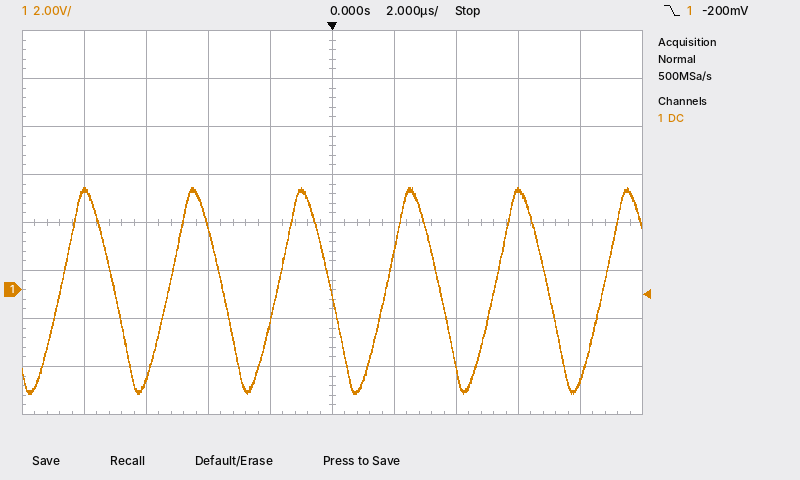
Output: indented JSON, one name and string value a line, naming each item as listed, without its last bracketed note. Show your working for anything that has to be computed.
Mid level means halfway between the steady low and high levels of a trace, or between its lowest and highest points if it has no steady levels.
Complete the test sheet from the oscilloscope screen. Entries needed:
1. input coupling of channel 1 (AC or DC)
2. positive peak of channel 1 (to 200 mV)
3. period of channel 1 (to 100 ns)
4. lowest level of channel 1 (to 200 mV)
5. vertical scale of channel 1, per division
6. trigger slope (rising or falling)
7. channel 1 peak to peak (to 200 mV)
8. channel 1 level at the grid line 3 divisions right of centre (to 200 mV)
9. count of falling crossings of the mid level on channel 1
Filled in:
{
  "input coupling of channel 1": "DC",
  "positive peak of channel 1": "4.2 V",
  "period of channel 1": "3.5 µs",
  "lowest level of channel 1": "-4.4 V",
  "vertical scale of channel 1, per division": "2 V",
  "trigger slope": "falling",
  "channel 1 peak to peak": "4.2 V − (-4.4 V) = 8.6 V",
  "channel 1 level at the grid line 3 divisions right of centre": "4.2 V",
  "count of falling crossings of the mid level on channel 1": "5"
}
